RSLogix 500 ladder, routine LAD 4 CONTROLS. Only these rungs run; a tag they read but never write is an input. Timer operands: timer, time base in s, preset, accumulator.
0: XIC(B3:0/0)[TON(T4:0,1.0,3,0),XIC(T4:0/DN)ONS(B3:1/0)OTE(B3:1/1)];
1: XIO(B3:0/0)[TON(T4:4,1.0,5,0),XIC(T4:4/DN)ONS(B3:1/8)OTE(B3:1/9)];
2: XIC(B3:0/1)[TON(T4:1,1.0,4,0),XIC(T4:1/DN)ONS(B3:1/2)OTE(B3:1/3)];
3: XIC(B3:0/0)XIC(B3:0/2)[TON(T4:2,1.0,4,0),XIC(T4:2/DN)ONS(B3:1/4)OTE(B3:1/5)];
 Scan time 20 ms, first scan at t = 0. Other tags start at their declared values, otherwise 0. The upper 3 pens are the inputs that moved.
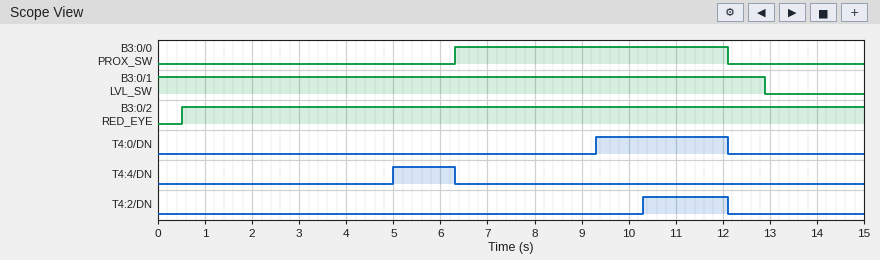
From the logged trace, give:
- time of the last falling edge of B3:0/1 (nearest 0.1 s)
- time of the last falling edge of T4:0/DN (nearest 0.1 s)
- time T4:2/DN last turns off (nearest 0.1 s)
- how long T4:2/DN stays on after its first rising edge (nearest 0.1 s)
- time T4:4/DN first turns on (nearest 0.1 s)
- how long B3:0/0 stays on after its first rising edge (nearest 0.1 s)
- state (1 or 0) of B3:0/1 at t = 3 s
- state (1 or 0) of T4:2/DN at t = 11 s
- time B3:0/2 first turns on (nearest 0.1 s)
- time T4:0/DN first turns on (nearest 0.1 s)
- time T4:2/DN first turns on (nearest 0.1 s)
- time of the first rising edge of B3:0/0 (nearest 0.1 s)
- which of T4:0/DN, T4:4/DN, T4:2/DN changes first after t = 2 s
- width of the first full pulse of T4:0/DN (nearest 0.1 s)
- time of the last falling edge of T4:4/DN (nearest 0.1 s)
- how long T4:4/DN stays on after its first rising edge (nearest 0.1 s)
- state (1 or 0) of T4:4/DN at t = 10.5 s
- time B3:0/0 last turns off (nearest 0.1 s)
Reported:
12.9 s
12.1 s
12.1 s
1.8 s
5.0 s
5.8 s
1
1
0.5 s
9.3 s
10.3 s
6.3 s
T4:4/DN
2.8 s
6.3 s
1.3 s
0
12.1 s
